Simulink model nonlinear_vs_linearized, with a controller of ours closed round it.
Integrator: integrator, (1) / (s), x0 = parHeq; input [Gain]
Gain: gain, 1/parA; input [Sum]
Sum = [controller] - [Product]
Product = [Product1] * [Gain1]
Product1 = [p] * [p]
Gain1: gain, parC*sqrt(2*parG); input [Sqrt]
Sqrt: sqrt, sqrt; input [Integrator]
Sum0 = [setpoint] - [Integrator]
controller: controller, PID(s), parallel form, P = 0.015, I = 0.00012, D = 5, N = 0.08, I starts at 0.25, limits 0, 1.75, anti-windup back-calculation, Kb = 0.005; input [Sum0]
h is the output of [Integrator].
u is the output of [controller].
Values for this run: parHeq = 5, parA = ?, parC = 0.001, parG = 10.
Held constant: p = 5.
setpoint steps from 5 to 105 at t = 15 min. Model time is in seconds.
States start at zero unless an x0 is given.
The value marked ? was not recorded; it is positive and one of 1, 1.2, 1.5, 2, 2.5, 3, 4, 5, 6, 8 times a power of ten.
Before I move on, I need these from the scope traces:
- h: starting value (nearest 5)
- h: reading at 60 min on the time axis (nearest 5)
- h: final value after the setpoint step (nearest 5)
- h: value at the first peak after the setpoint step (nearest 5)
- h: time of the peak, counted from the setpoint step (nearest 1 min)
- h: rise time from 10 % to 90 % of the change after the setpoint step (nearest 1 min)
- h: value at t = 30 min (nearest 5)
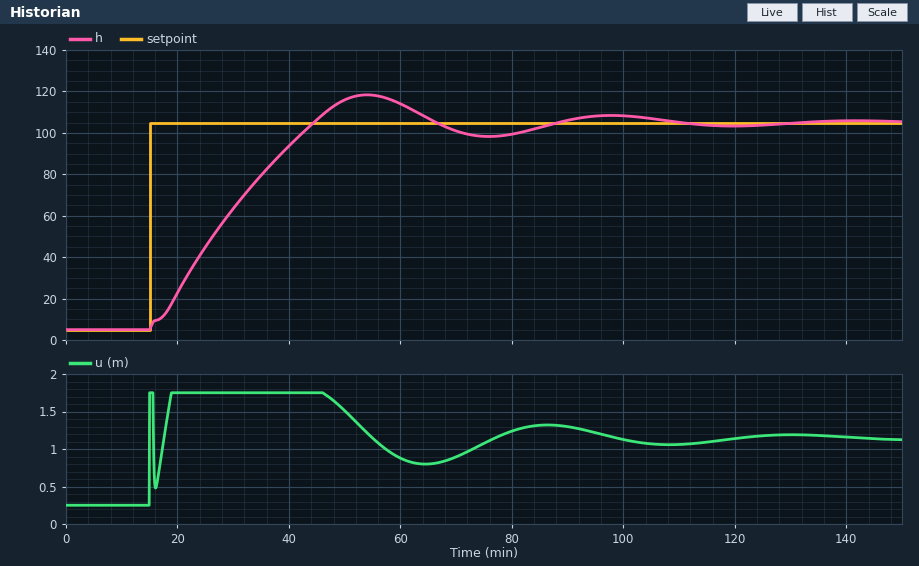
5
115
105
120
39 min
22 min
65
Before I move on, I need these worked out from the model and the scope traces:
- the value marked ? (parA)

15
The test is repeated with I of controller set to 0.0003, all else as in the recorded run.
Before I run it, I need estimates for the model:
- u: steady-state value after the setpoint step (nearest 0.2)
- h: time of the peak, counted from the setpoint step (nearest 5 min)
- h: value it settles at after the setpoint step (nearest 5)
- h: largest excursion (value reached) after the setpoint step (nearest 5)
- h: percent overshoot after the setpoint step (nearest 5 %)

1.2
35 min
105
115
10 %
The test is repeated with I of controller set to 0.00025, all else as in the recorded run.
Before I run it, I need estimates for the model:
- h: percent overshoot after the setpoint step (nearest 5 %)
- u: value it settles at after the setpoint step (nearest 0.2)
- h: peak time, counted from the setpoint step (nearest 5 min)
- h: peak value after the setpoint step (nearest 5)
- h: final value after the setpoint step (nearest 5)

10 %
1.2
35 min
115
105
